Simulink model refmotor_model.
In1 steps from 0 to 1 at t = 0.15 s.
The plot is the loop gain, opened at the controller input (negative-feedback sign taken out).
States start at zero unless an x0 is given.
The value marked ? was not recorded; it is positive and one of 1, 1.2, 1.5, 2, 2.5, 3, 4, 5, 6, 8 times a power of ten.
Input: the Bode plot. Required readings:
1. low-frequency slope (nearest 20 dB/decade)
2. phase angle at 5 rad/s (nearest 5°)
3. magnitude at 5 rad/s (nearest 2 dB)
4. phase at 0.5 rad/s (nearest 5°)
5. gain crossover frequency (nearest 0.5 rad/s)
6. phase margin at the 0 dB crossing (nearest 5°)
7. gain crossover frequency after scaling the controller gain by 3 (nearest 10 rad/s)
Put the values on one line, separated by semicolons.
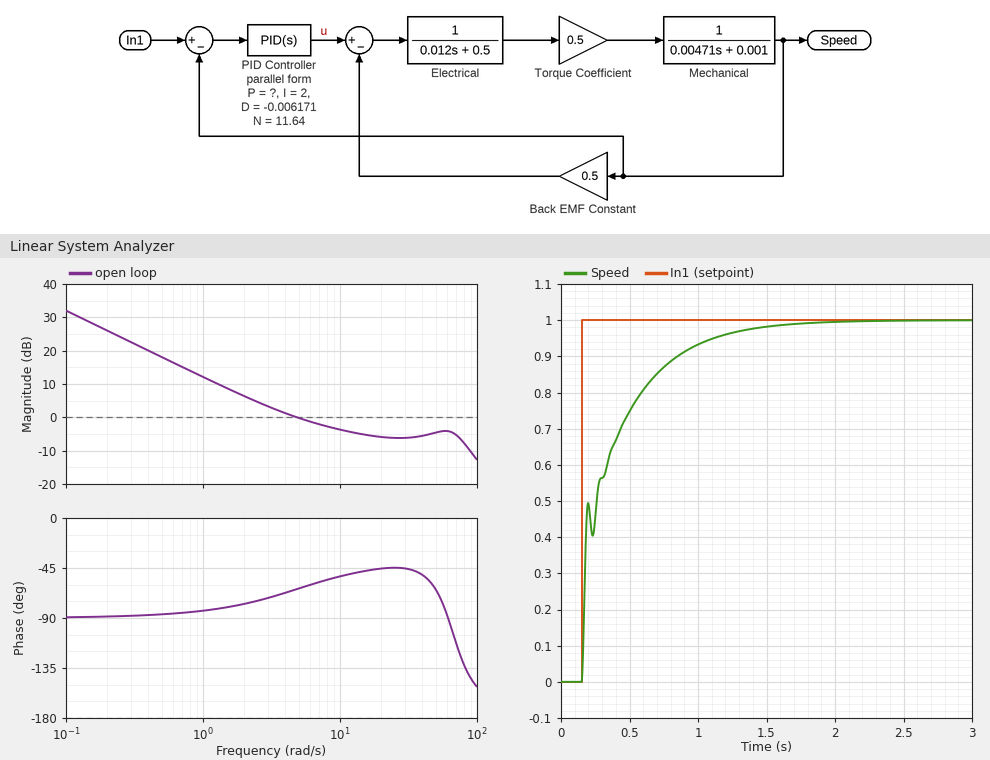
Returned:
-20 dB/decade; -65°; 0 dB; -85°; 5.0 rad/s; 115°; 90 rad/s
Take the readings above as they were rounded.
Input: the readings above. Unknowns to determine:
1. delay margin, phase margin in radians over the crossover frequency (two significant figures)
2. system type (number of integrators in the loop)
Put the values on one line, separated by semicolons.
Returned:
0.40 s; 1
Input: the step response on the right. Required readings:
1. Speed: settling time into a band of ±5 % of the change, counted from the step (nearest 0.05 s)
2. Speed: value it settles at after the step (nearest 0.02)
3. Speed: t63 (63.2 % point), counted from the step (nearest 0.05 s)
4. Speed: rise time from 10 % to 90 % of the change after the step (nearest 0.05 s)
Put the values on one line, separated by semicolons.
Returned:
0.95 s; 1.00; 0.20 s; 0.70 s
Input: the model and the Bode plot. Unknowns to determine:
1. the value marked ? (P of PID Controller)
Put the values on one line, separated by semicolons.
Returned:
0.25
